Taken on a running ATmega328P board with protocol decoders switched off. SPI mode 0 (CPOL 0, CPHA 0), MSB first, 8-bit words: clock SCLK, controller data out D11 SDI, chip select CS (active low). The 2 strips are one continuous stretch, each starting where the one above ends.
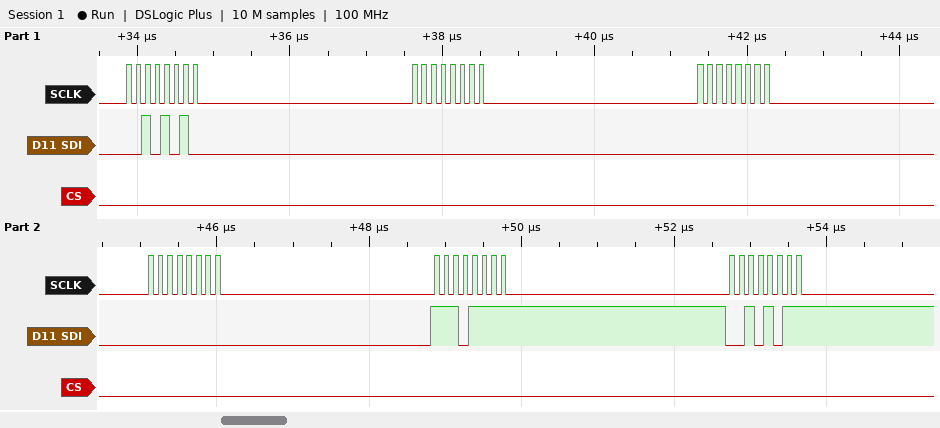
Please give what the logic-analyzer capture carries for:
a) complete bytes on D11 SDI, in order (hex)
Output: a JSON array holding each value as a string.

["0x2A 0x00 0x00 0x00 0xEF 0x2B"]
